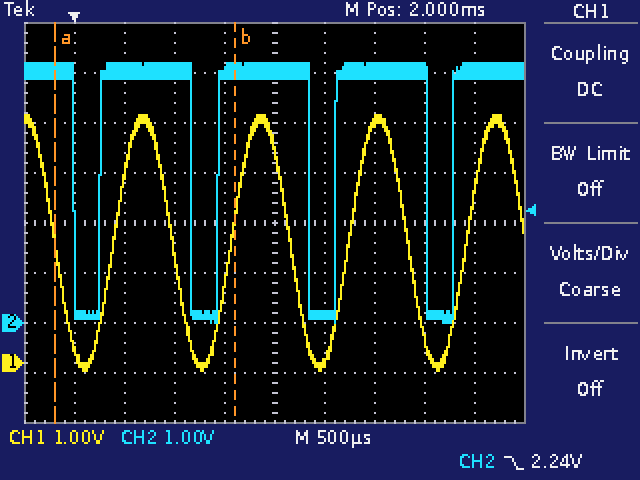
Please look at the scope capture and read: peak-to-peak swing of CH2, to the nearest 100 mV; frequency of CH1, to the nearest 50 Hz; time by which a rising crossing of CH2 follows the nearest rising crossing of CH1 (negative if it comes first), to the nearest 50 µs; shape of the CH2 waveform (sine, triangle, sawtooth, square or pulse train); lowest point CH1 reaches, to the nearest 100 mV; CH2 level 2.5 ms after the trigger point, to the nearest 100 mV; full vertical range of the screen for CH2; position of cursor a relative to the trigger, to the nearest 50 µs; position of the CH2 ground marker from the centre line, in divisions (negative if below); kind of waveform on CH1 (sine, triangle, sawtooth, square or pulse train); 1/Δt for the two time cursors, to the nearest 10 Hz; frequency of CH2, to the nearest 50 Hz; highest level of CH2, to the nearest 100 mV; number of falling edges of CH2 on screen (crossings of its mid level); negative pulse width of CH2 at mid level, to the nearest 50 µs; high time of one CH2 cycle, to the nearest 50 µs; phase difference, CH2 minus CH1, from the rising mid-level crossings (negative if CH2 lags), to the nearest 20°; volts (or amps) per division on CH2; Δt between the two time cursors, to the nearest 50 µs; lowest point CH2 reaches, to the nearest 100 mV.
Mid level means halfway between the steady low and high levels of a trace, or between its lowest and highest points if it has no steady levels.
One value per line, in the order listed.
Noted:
5.2 V
850 Hz
-150 µs
pulse train
-200 mV
200 mV
8 V
-200 µs
-2.0 div
sine
560 Hz
850 Hz
5.2 V
4
250 µs
900 µs
+40°
1 V
1.80 ms
0.0 V
